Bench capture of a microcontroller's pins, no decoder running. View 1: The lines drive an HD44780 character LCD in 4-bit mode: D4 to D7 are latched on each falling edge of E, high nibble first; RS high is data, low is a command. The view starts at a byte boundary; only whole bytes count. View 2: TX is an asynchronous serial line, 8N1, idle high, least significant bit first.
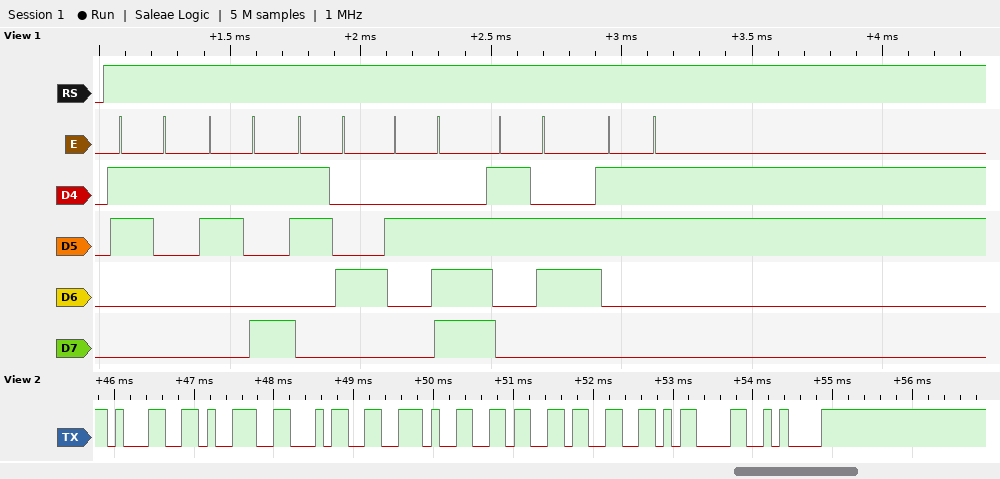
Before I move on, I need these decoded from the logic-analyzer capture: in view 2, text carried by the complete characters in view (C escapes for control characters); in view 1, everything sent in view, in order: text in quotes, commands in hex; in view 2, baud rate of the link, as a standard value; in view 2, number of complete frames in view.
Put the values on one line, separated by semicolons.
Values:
"194.63\r\n"; "194.63"; 9600 baud; 8
